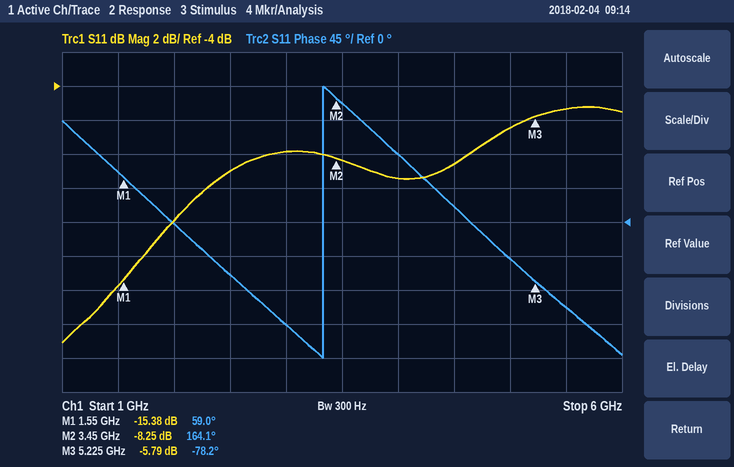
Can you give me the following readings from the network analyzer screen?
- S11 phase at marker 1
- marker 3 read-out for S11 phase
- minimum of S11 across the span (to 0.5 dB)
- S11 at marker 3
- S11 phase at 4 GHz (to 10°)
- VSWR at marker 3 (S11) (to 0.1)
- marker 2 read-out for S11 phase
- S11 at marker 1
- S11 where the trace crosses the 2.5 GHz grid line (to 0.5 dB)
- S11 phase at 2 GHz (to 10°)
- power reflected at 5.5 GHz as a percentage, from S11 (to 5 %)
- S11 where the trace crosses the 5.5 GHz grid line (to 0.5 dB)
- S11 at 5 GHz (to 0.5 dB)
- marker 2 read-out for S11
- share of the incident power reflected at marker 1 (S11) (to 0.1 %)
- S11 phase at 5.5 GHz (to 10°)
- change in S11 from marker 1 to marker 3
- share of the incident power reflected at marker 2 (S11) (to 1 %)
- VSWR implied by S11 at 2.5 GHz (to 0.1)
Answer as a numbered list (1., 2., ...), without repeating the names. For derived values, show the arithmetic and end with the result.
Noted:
1. 59.0°
2. -78.2°
3. -19.0 dB
4. -5.79 dB
5. 90°
6. (1 + 0.5135)/(1 − 0.5135) ≈ 3.1
7. 164.1°
8. -15.38 dB
9. -9.0 dB
10. 0°
11. 10^(-5.5/10) ≈ 28.2 %, so 30 % to the nearest 5 %
12. -5.5 dB
13. -6.5 dB
14. -8.25 dB
15. 10^(-15.38/10) ≈ 2.9 %
16. -110°
17. -5.79 − (-15.38) = 9.59 dB
18. 10^(-8.25/10) ≈ 15 %
19. |Γ| = 10^(-9/20) = 0.3548; VSWR = (1 + 0.3548)/(1 − 0.3548) ≈ 2.1
